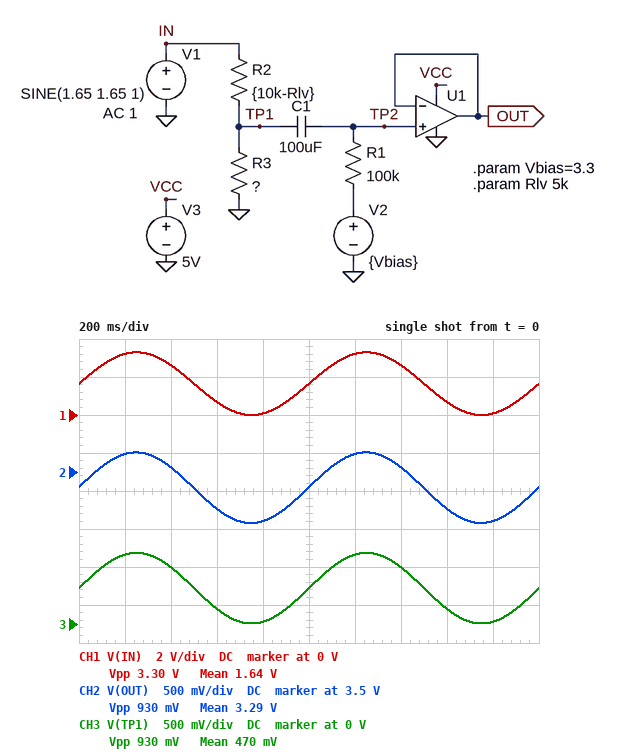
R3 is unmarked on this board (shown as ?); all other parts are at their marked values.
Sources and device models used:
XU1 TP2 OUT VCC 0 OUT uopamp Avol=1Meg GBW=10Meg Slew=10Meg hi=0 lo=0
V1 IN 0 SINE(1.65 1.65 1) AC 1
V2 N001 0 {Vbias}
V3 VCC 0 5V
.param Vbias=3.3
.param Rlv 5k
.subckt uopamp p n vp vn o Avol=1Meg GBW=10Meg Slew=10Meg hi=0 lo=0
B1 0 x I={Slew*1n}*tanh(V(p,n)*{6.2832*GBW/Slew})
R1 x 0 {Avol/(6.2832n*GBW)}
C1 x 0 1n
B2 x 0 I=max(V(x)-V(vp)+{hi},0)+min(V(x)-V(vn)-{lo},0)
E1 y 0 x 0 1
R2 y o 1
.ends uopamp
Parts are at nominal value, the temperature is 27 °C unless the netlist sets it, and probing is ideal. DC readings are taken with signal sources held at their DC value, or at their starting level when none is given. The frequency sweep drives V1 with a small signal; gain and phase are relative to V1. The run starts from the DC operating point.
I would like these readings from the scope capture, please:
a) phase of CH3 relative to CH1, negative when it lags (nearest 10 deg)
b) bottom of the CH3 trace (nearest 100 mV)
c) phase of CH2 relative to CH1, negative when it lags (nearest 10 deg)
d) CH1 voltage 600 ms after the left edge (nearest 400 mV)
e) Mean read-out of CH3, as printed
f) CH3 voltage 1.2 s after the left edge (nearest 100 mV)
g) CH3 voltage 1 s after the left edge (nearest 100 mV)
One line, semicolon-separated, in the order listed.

0 deg; 0 V; 0 deg; 800 mV; 470 mV; 900 mV; 500 mV
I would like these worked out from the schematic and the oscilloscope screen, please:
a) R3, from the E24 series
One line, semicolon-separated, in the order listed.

2 kΩ
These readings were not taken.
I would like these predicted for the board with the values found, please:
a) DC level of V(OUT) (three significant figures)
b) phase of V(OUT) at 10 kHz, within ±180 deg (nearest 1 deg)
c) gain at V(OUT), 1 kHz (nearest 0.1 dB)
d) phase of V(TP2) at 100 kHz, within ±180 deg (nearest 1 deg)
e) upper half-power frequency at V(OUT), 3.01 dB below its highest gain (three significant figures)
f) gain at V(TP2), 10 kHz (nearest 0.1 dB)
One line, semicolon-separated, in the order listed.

3.30 V; 0 deg; -11.0 dB; 0 deg; 10.0 MHz; -11.0 dB
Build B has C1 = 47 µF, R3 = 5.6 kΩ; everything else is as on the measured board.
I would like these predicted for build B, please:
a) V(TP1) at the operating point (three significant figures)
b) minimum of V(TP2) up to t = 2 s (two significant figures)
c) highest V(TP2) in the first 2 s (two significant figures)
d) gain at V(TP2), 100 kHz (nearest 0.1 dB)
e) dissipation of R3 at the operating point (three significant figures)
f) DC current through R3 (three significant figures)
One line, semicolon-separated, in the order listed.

872 mV; 2.4 V; 4.1 V; -5.8 dB; 136 µW; 156 µA
